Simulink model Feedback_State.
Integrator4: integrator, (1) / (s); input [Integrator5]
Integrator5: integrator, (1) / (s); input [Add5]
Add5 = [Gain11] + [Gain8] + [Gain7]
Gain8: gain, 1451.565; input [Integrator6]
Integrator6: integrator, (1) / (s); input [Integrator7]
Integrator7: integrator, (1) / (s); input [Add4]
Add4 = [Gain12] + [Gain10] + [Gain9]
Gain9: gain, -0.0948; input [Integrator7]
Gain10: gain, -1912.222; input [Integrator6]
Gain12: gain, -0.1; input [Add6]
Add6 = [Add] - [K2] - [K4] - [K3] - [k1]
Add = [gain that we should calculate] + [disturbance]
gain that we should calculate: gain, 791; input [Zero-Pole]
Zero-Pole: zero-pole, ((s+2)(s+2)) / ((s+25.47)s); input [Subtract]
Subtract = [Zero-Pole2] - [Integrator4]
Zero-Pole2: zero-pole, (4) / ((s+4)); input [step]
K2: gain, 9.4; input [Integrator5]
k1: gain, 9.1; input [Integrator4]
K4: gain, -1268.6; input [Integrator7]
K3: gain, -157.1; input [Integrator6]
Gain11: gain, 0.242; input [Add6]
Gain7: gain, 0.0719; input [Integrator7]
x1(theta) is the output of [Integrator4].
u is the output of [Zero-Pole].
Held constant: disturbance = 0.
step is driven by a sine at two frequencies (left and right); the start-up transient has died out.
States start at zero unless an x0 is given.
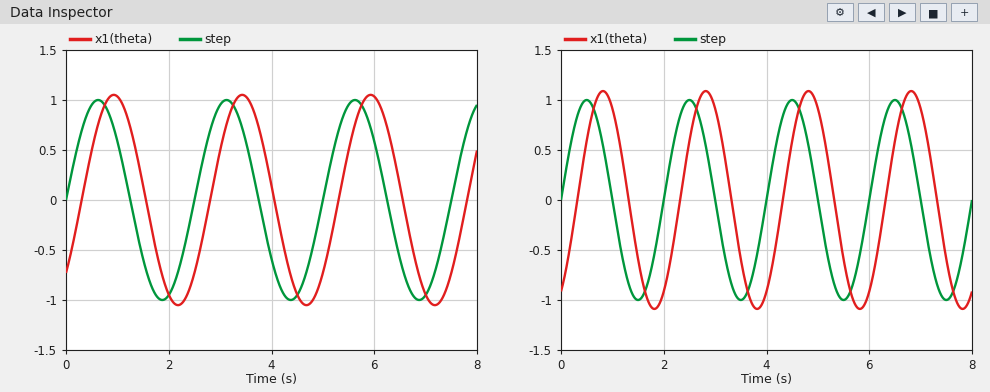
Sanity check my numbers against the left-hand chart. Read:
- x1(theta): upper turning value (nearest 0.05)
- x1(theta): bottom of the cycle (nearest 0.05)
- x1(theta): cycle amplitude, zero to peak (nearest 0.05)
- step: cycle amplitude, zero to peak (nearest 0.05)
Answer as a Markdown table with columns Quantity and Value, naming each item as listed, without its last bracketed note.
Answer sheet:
| Quantity | Value |
|---|---|
| x1(theta): upper turning value | 1.05 |
| x1(theta): bottom of the cycle | -1.05 |
| x1(theta): cycle amplitude, zero to peak | 1.05 |
| step: cycle amplitude, zero to peak | 1.00 |
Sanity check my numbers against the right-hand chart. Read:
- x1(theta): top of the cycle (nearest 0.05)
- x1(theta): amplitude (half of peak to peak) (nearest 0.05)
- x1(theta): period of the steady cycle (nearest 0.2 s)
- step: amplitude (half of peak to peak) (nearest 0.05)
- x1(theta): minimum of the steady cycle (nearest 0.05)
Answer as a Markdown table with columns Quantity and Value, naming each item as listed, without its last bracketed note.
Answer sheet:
| Quantity | Value |
|---|---|
| x1(theta): top of the cycle | 1.10 |
| x1(theta): amplitude (half of peak to peak) | 1.10 |
| x1(theta): period of the steady cycle | 2.0 s |
| step: amplitude (half of peak to peak) | 1.00 |
| x1(theta): minimum of the steady cycle | -1.10 |
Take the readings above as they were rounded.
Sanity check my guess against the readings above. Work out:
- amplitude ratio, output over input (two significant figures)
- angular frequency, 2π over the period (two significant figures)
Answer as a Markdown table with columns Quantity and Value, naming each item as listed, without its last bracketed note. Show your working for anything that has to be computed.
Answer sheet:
| Quantity | Value |
|---|---|
| amplitude ratio, output over input | 1.1 / 1 = 1.1 |
| angular frequency, 2π over the period | 2π / 2 = 3.1 rad/s |
